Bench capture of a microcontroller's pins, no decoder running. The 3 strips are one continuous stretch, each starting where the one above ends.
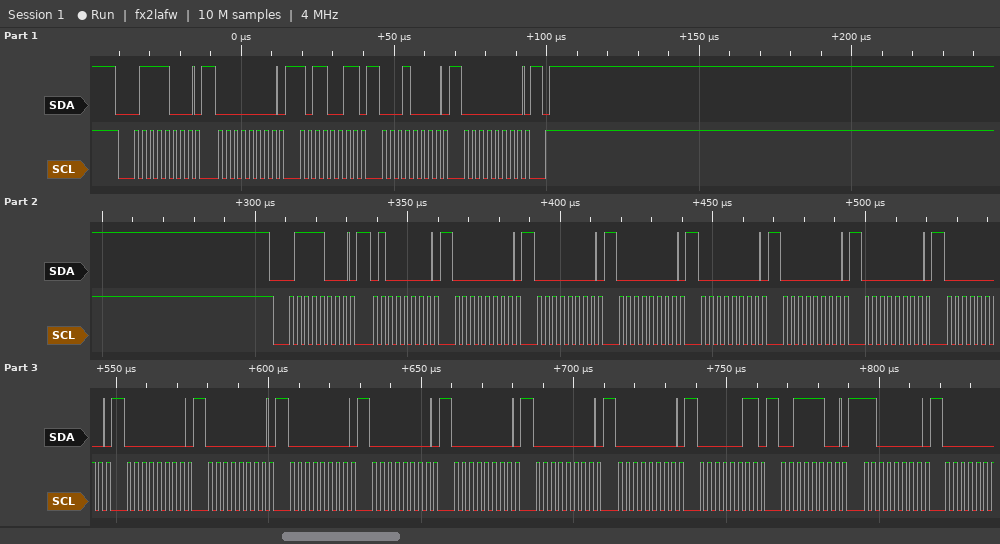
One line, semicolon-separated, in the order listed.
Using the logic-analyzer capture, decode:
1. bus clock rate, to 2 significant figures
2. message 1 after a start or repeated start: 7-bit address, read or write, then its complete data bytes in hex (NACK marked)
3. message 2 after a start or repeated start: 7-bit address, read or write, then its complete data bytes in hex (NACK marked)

400 kHz; 0x3C write: 00 B3 10 00; 0x3C write: 40 00 00 00 00 00 00 00 00 00 00 00 00 00 00 03 3C C0
